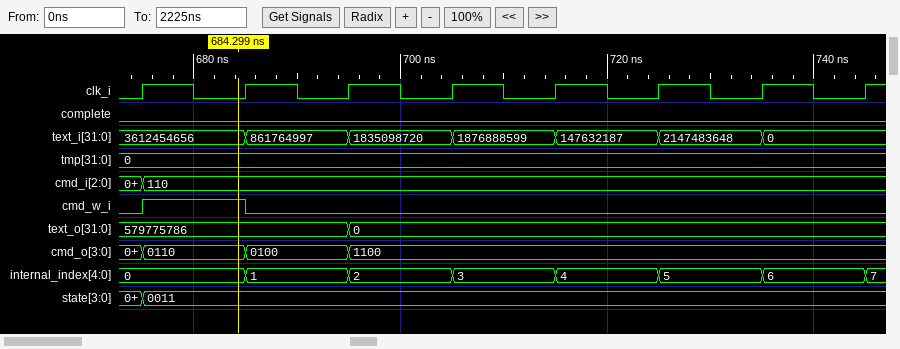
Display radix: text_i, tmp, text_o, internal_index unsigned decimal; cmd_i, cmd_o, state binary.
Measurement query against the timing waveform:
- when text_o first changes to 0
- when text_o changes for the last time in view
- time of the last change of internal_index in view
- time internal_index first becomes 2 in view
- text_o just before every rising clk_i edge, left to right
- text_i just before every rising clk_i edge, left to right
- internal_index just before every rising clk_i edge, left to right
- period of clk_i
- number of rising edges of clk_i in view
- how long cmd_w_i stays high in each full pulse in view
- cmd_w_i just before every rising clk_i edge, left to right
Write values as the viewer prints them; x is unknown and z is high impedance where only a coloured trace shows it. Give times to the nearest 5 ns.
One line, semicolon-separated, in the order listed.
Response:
695 ns; 695 ns; 745 ns; 695 ns; 579775786, 579775786, 579775786, 0, 0, 0, 0, 0; 3612454656, 3612454656, 861764997, 1835098720, 1876888599, 147632187, 2147483648, 0; 0, 0, 1, 2, 3, 4, 5, 6; 10 ns; 8; 10 ns; 0 1 0 0 0 0 0 0
